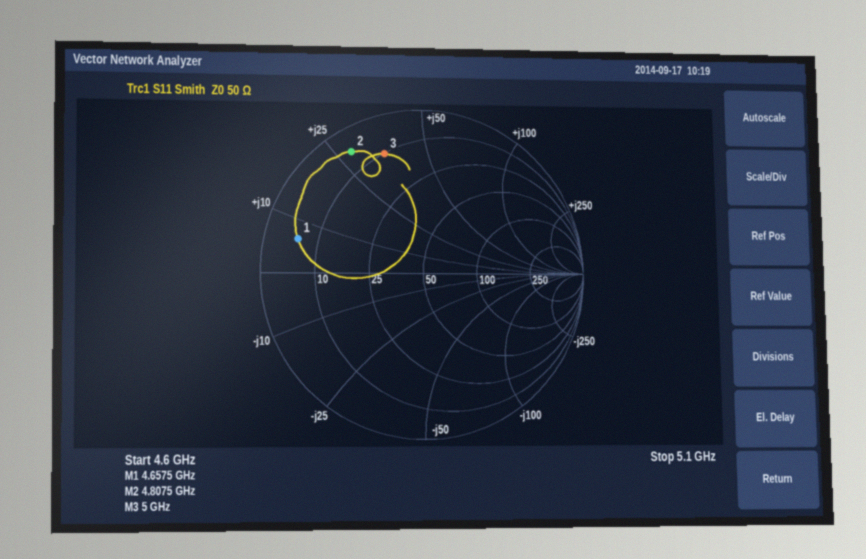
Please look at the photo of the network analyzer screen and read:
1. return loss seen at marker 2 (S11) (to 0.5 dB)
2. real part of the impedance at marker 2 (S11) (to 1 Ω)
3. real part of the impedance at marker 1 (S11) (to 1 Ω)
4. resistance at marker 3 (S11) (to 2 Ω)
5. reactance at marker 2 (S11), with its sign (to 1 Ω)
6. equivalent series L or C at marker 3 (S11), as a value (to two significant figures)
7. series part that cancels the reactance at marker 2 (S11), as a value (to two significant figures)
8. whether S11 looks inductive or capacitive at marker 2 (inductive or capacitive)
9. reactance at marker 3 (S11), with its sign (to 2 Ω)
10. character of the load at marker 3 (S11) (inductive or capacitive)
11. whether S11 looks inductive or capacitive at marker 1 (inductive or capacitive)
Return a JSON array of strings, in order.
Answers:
["1.5 dB", "5 Ω", "6 Ω", "10 Ω", "+28 Ω", "1.1 nH", "1.2 pF", "inductive", "+36 Ω", "inductive", "inductive"]
